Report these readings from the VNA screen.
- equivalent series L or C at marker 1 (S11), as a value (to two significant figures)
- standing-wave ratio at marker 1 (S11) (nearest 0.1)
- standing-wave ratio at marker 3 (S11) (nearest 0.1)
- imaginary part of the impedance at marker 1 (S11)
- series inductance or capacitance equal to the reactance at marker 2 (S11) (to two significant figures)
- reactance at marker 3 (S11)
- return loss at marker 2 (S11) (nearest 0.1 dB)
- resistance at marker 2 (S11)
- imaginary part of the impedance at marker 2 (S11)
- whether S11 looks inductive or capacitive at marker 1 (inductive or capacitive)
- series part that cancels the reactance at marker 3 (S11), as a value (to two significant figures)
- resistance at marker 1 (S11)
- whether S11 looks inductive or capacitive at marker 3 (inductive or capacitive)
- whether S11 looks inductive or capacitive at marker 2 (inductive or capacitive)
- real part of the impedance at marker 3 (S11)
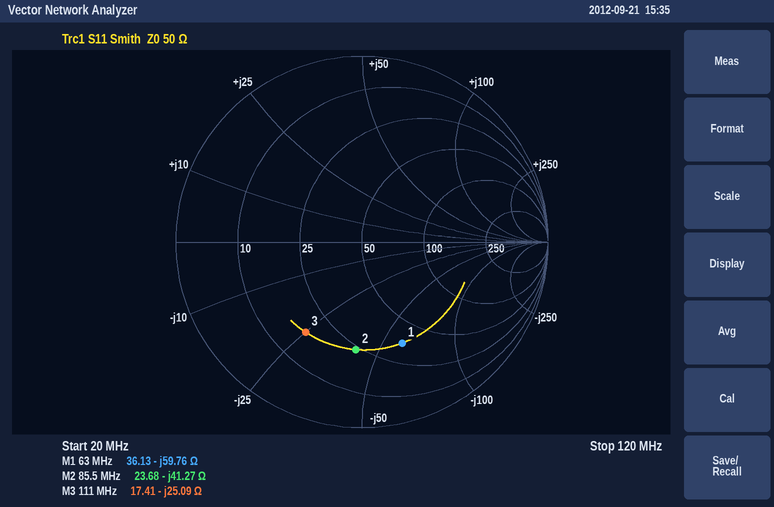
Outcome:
42 pF
3.8
3.7
-59.76 Ω
45 pF
-25.09 Ω
4.7 dB
23.68 Ω
-41.27 Ω
capacitive
36 nH
36.13 Ω
capacitive
capacitive
17.41 Ω
